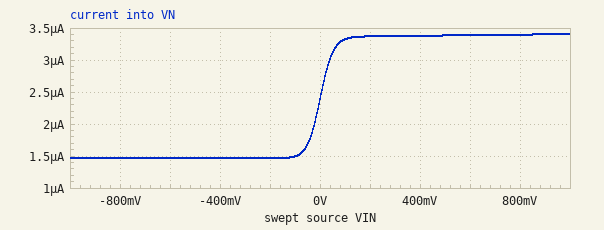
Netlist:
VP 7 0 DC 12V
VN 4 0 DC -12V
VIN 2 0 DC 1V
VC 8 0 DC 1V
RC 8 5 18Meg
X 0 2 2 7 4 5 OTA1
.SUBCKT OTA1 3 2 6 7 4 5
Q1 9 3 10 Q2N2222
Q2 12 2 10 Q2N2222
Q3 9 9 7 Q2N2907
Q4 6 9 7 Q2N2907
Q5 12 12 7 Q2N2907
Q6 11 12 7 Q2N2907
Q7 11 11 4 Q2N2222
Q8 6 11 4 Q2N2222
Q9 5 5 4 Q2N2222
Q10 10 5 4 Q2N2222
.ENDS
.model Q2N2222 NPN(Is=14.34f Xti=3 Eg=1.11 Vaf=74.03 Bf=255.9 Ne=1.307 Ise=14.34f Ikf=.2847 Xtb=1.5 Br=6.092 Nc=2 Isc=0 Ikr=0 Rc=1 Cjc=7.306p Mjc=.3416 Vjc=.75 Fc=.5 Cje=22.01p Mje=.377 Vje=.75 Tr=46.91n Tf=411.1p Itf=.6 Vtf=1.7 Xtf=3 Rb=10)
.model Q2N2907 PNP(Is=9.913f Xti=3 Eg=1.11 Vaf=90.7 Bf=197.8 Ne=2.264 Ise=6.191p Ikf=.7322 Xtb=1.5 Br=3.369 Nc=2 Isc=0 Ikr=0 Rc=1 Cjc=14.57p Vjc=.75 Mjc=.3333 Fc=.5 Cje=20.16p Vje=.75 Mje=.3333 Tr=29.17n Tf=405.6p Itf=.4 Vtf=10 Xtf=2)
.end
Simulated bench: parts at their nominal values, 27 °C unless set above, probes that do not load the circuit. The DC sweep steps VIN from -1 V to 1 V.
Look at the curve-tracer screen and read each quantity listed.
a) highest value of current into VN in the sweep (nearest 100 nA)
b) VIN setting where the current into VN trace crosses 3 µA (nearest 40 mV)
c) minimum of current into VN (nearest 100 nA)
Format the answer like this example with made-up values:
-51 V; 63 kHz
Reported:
3.4 µA; 40 mV; 1.5 µA
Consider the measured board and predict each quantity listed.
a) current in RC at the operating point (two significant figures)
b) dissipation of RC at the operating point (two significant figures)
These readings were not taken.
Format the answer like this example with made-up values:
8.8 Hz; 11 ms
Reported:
700 nA; 8.7 µW
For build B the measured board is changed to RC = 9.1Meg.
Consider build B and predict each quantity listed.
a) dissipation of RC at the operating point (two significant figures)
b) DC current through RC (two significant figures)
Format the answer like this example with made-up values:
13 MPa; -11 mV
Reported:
17 µW; 1.4 µA
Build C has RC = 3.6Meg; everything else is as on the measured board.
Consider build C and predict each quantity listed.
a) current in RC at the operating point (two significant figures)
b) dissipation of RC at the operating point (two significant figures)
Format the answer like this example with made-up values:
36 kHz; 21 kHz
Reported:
3.5 µA; 43 µW
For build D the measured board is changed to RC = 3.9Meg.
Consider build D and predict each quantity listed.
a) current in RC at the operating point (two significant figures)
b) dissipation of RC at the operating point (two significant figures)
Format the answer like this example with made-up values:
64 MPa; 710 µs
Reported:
3.2 µA; 40 µW
